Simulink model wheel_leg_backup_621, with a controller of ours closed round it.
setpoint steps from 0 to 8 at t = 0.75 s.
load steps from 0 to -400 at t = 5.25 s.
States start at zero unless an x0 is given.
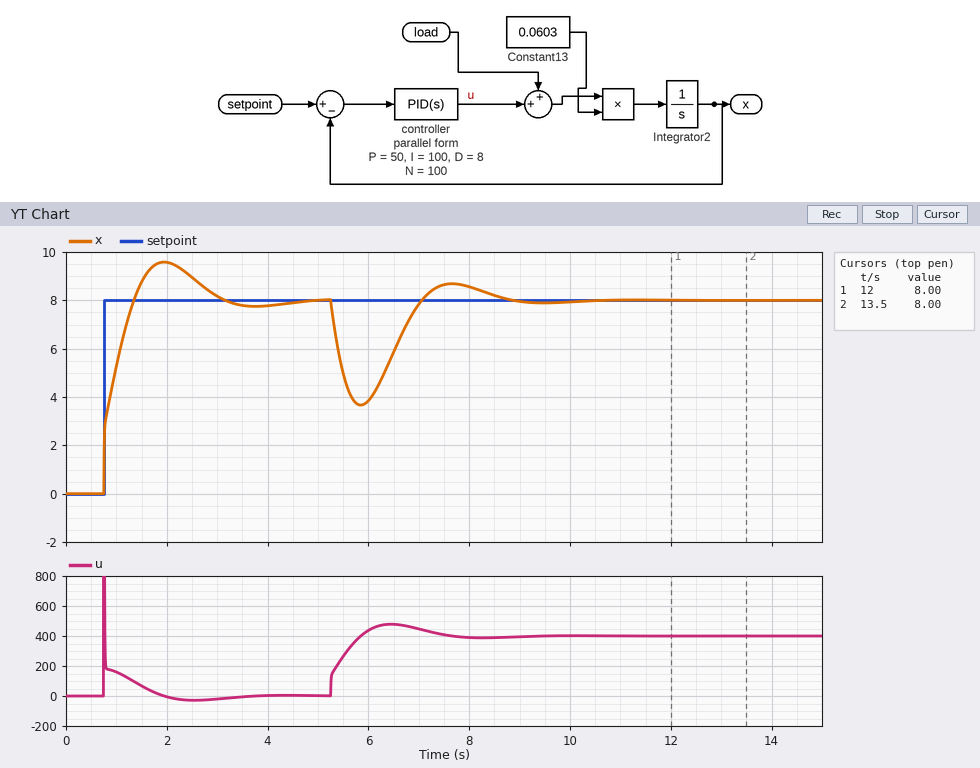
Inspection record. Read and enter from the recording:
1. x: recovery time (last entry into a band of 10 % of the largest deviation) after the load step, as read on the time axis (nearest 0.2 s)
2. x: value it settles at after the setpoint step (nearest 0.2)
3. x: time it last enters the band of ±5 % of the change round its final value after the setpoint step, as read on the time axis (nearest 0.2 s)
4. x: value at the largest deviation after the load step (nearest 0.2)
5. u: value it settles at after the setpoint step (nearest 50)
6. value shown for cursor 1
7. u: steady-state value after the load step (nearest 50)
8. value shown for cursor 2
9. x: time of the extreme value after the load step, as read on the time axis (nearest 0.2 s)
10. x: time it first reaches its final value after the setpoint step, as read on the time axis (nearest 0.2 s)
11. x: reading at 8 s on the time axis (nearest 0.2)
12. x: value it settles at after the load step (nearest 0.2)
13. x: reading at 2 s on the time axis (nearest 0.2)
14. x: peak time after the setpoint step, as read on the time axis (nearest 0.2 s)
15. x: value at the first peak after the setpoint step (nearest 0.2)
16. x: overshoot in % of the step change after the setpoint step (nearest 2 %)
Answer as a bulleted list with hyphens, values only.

- 8.2 s
- 8.0
- 2.8 s
- 3.6
- 0
- 8.00
- 400
- 8.00
- 5.8 s
- 1.4 s
- 8.6
- 8.0
- 9.6
- 2.0 s
- 9.6
- 20 %
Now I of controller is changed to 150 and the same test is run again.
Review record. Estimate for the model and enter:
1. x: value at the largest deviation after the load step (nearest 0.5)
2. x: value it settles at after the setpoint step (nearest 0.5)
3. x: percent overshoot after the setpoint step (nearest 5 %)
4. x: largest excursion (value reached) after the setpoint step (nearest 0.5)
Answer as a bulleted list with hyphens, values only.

- 4.0
- 8.0
- 25 %
- 10.0
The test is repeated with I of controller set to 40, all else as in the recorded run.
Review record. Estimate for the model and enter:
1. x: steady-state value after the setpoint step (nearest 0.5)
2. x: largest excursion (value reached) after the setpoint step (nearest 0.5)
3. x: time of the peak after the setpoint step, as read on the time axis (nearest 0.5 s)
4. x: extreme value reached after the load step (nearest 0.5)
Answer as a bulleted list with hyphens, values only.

- 8.0
- 9.0
- 2.5 s
- 2.5
